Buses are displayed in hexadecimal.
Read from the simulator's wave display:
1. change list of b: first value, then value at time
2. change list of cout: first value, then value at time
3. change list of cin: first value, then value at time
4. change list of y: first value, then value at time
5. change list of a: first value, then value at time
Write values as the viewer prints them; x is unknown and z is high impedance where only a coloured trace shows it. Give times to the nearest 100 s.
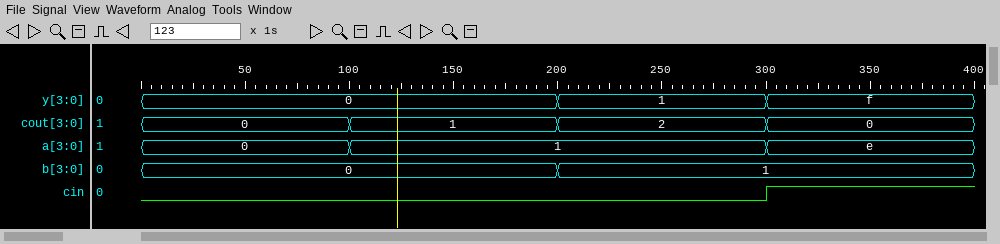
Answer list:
0, 1 at 200 s
0, 1 at 100 s, 2 at 200 s, 0 at 300 s
0, 1 at 300 s
0, 1 at 200 s, f at 300 s
0, 1 at 100 s, e at 300 s
